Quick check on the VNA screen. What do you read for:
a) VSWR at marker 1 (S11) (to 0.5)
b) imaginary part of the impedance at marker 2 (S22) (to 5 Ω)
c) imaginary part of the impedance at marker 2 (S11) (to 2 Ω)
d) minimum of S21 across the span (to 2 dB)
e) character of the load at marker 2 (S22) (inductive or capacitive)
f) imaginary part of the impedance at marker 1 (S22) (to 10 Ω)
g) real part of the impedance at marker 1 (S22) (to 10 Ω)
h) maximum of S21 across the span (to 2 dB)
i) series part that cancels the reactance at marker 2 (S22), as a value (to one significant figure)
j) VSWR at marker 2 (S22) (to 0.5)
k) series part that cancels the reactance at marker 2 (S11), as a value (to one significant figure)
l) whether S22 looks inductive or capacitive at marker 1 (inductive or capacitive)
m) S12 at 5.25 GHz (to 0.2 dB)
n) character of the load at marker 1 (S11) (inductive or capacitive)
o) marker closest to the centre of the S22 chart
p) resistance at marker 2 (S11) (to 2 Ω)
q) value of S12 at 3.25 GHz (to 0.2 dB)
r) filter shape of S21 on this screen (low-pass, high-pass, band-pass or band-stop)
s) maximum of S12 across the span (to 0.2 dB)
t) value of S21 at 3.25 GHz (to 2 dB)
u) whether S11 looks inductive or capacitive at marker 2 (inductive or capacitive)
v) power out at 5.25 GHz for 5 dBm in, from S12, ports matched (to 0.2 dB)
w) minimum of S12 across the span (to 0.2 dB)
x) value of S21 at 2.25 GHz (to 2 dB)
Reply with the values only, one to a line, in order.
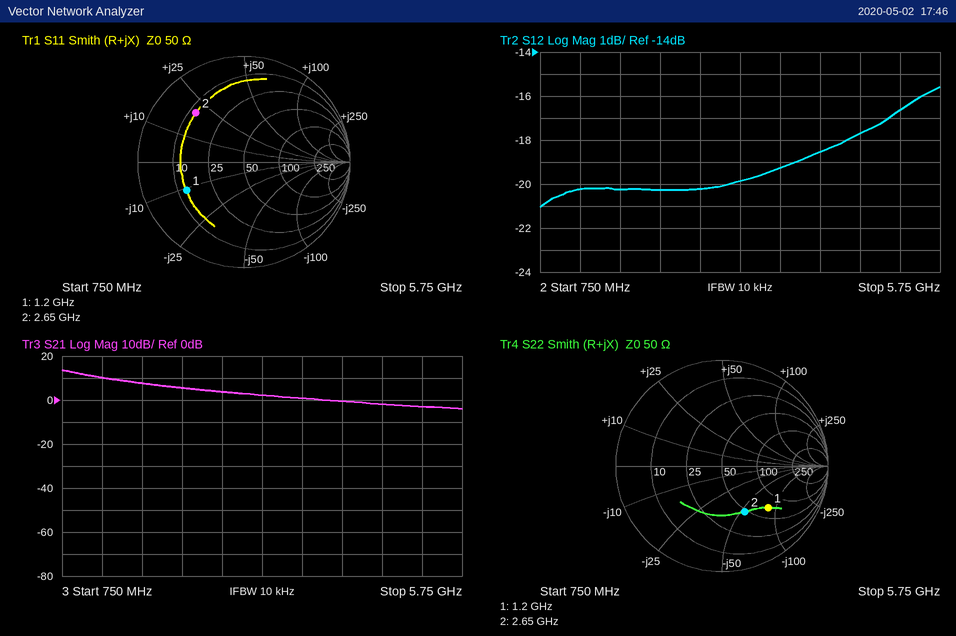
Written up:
4.0
-55 Ω
+20 Ω
-4 dB
capacitive
-80 Ω
70 Ω
14 dB
3 nH
3.0
3 pF
capacitive
-16.6 dB
capacitive
marker 2
12 Ω
-19.8 dB
low-pass
-15.6 dB
2 dB
inductive
-11.6 dBm
-21.0 dB
6 dB
